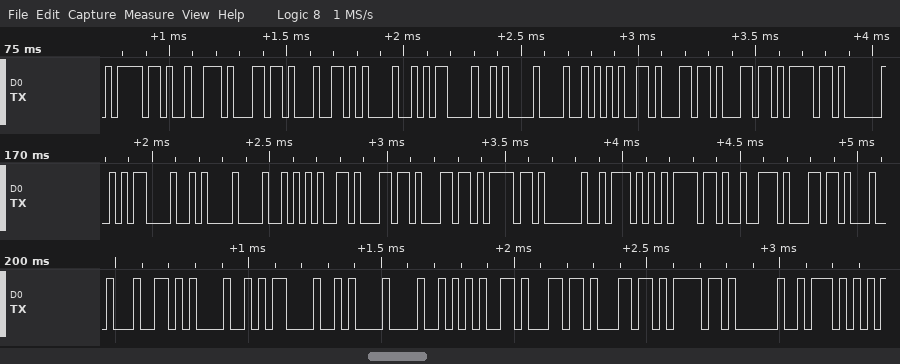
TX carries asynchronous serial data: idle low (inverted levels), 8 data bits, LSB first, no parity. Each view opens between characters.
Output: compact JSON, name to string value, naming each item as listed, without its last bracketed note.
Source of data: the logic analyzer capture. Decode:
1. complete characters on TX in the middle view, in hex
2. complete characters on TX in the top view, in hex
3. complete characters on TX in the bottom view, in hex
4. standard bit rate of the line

{"complete characters on TX in the middle view, in hex": "E5, EB, 6F, 35, 27, 27, 21, BF, 51, 21, 1B, 27", "complete characters on TX in the top view, in hex": "21, 1B, 27, 37, BD, E5, EB, 6F, 35, 27, 27, 21", "complete characters on TX in the bottom view, in hex": "37, BD, E5, EB, 6F, 35, 27, 27, 21, BF, 51", "standard bit rate of the line": "38400 baud"}
